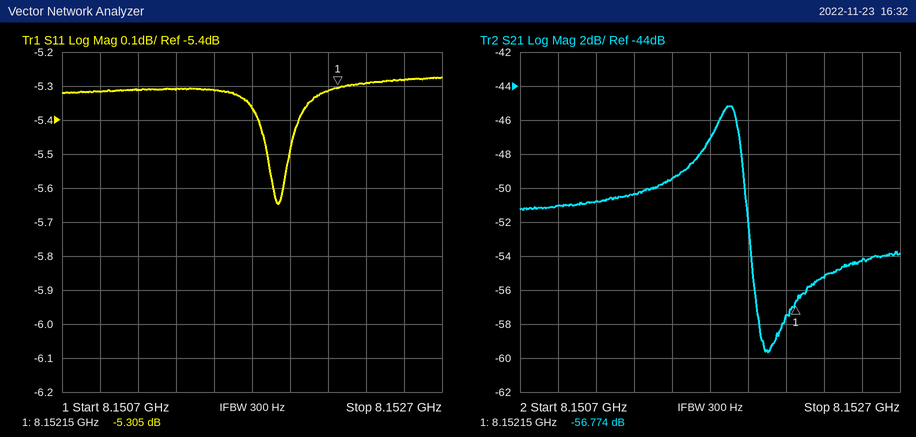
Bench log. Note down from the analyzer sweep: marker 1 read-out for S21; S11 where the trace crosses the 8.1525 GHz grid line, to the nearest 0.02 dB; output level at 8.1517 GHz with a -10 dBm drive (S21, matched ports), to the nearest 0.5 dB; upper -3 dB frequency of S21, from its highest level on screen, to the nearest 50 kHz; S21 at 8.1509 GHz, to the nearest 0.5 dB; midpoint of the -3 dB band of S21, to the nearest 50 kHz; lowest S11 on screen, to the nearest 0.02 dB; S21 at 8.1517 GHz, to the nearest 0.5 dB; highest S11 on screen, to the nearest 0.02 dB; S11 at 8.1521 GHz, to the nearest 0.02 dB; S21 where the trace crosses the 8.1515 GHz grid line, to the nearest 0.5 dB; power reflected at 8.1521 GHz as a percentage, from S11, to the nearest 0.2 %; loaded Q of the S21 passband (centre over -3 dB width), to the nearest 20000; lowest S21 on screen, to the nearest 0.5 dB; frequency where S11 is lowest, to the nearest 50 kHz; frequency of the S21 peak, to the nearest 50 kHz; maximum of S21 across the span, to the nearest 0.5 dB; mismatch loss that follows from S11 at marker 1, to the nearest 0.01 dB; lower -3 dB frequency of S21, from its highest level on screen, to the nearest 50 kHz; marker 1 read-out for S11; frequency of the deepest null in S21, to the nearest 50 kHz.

-56.774 dB
-5.28 dB
-57.0 dBm
8.15185 GHz
-51.0 dB
8.15175 GHz
-5.64 dB
-47.0 dB
-5.28 dB
-5.32 dB
-49.5 dB
29.4 %
40000
-59.5 dB
8.15185 GHz
8.15180 GHz
-45.0 dB
1.52 dB
8.15165 GHz
-5.305 dB
8.15200 GHz
